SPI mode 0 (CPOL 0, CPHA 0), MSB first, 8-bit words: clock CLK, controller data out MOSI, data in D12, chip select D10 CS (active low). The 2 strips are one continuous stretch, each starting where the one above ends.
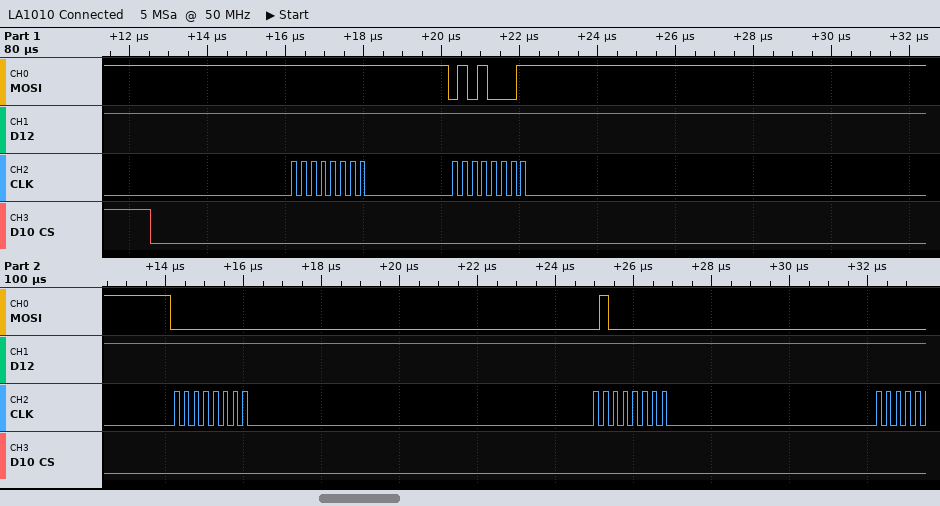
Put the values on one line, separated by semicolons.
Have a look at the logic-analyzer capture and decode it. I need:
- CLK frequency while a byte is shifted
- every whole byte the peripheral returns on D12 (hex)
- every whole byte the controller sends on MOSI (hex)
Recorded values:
4 MHz; FF FF FF FF; FF 51 00 40
